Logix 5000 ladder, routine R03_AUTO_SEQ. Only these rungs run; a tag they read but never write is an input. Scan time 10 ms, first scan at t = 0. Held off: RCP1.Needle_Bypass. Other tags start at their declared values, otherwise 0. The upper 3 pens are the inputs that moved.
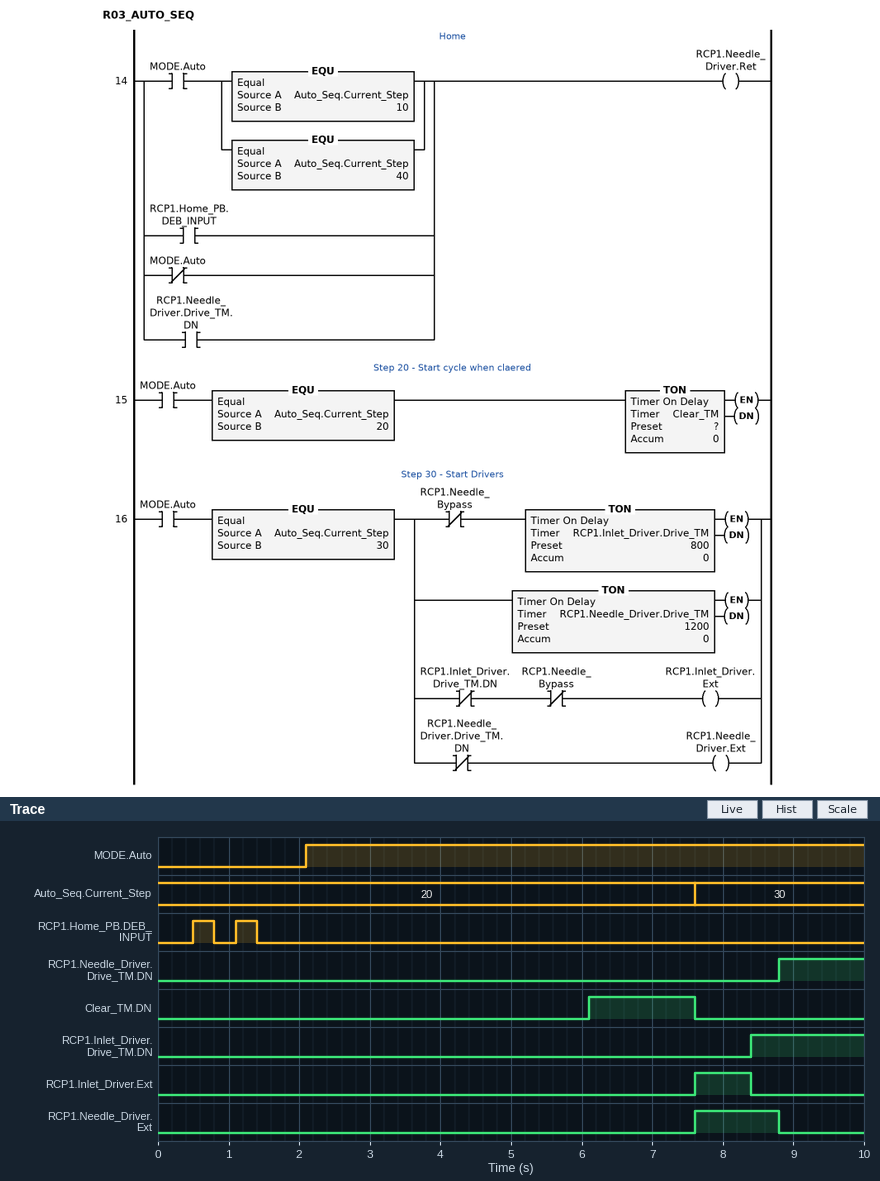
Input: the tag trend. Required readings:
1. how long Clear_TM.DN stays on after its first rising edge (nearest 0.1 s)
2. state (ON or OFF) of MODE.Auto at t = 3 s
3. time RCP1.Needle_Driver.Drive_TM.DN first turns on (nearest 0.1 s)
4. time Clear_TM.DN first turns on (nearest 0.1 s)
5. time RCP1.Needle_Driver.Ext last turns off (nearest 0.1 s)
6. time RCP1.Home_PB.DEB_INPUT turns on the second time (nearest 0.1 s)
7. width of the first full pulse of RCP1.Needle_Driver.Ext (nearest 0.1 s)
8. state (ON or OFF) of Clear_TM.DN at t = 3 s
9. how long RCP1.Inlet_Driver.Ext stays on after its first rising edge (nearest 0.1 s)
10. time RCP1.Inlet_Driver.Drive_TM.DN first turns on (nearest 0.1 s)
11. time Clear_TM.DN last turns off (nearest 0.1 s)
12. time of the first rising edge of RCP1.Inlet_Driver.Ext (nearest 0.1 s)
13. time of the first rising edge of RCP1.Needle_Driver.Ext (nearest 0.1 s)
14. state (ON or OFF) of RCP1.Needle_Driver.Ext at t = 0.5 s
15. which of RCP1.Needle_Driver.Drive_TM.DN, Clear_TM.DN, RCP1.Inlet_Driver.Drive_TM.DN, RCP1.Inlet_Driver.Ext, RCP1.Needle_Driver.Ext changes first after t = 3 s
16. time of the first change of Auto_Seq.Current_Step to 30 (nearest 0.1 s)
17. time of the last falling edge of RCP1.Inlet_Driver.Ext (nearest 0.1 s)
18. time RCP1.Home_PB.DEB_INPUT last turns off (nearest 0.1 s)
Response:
1.5 s
ON
8.8 s
6.1 s
8.8 s
1.1 s
1.2 s
OFF
0.8 s
8.4 s
7.6 s
7.6 s
7.6 s
OFF
Clear_TM.DN
7.6 s
8.4 s
1.4 s
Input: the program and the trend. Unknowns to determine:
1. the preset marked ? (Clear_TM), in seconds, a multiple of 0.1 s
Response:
4.0 s
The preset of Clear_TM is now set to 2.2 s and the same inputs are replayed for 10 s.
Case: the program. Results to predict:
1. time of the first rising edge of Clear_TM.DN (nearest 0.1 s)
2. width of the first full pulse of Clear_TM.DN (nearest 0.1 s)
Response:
4.3 s
3.3 s
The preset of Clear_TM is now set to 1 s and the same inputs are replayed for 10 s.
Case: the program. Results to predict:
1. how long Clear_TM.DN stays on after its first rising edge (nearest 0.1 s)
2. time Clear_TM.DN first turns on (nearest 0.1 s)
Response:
4.5 s
3.1 s
